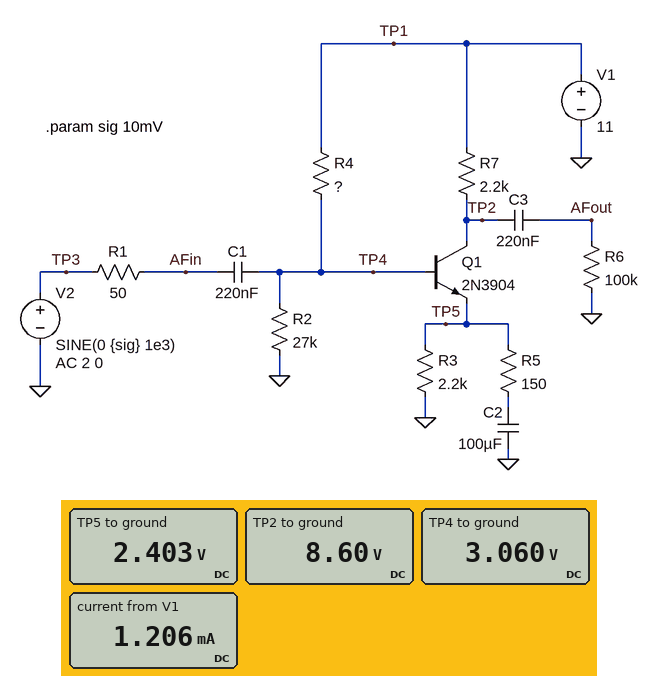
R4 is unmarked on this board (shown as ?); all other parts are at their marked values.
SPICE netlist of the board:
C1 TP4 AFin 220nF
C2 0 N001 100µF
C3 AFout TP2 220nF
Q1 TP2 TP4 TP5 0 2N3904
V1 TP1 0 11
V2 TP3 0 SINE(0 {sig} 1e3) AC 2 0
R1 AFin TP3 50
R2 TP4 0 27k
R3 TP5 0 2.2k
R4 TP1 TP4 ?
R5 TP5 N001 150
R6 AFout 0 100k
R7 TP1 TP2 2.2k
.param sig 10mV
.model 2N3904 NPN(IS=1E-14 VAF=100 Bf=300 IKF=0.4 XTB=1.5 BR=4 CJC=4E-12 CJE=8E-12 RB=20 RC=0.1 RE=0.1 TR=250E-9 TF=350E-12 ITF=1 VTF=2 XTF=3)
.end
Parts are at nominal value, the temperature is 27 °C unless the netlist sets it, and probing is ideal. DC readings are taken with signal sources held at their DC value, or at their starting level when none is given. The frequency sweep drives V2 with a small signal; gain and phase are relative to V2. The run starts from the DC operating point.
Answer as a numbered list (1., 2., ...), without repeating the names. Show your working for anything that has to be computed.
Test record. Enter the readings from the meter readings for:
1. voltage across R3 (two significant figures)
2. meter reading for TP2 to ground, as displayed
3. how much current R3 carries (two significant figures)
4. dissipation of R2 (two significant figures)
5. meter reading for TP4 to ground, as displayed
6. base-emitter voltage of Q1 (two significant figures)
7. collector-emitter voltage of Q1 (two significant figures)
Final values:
1. 2.403 V = 2.4 V
2. 8.60 V
3. (2.403 V) / 2.2 kΩ = 1.1 mA
4. (3.06 V)^2 / 27 kΩ = 350 µW
5. 3.060 V
6. 3.06 V - 2.403 V = 660 mV
7. 8.6 V - 2.403 V = 6.2 V
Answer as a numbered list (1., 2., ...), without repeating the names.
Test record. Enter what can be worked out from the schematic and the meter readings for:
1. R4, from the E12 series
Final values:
1. 68 kΩ
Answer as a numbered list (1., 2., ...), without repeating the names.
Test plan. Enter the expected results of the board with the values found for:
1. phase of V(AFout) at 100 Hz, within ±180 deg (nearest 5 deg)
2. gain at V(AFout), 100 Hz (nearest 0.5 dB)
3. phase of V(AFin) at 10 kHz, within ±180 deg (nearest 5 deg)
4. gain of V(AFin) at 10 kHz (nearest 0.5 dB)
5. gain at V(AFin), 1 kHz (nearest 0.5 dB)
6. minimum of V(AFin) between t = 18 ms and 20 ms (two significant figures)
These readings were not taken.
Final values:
1. -145 deg
2. 21.0 dB
3. 0 deg
4. 0 dB
5. 0 dB
6. -10 mV
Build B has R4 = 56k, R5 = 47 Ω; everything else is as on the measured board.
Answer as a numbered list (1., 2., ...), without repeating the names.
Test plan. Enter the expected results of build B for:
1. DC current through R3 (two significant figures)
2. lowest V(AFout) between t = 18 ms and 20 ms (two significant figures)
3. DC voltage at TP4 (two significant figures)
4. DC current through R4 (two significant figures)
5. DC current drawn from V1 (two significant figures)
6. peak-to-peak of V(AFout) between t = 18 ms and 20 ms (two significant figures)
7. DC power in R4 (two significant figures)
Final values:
1. 1.3 mA
2. -320 mV
3. 3.5 V
4. 130 µA
5. 1.4 mA
6. 640 mV
7. 1.0 mW
